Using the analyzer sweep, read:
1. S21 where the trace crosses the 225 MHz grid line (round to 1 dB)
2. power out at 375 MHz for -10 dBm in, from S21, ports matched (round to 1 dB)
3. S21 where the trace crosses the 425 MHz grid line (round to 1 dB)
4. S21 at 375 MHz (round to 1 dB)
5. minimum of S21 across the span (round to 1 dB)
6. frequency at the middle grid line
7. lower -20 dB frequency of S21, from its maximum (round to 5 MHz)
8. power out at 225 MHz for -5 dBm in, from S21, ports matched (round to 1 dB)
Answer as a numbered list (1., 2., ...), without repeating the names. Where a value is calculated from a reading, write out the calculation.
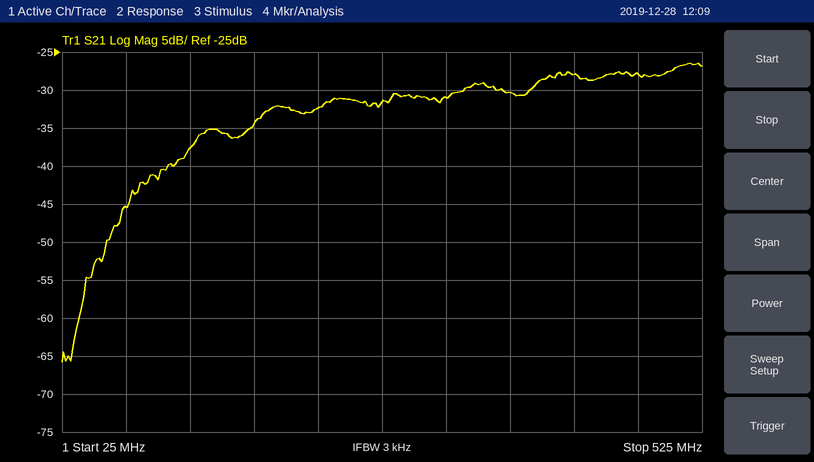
1. -32 dB
2. -10 dBm + (-30 dB) = -40 dBm
3. -28 dB
4. -30 dB
5. -66 dB
6. 275 MHz
7. 70 MHz
8. -5 dBm + (-32 dB) = -37 dBm
